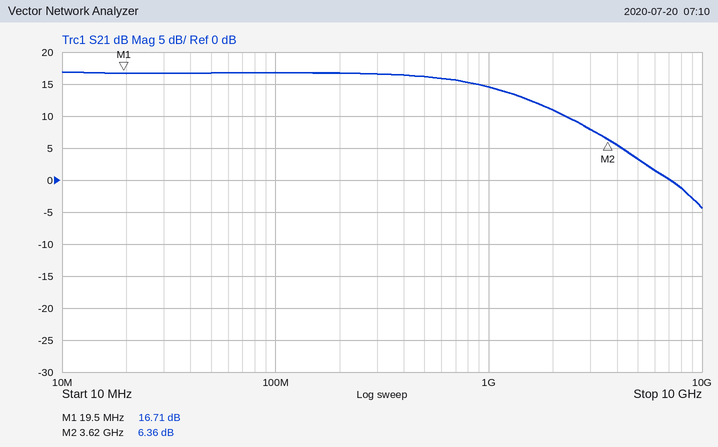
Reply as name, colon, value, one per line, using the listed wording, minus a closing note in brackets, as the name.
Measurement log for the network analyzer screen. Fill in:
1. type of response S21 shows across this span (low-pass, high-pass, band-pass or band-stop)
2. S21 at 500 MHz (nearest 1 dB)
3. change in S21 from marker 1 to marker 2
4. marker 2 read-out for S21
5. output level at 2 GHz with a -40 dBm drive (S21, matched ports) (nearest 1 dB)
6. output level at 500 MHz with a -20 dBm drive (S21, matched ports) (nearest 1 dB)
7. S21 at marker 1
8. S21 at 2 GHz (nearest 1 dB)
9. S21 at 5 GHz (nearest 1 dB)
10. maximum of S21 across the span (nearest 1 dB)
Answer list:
type of response S21 shows across this span: low-pass
S21 at 500 MHz: 16 dB
change in S21 from marker 1 to marker 2: -10.35 dB
marker 2 read-out for S21: 6.36 dB
output level at 2 GHz with a -40 dBm drive (S21, matched ports): -29 dBm
output level at 500 MHz with a -20 dBm drive (S21, matched ports): -4 dBm
S21 at marker 1: 16.71 dB
S21 at 2 GHz: 11 dB
S21 at 5 GHz: 3 dB
maximum of S21 across the span: 17 dB
